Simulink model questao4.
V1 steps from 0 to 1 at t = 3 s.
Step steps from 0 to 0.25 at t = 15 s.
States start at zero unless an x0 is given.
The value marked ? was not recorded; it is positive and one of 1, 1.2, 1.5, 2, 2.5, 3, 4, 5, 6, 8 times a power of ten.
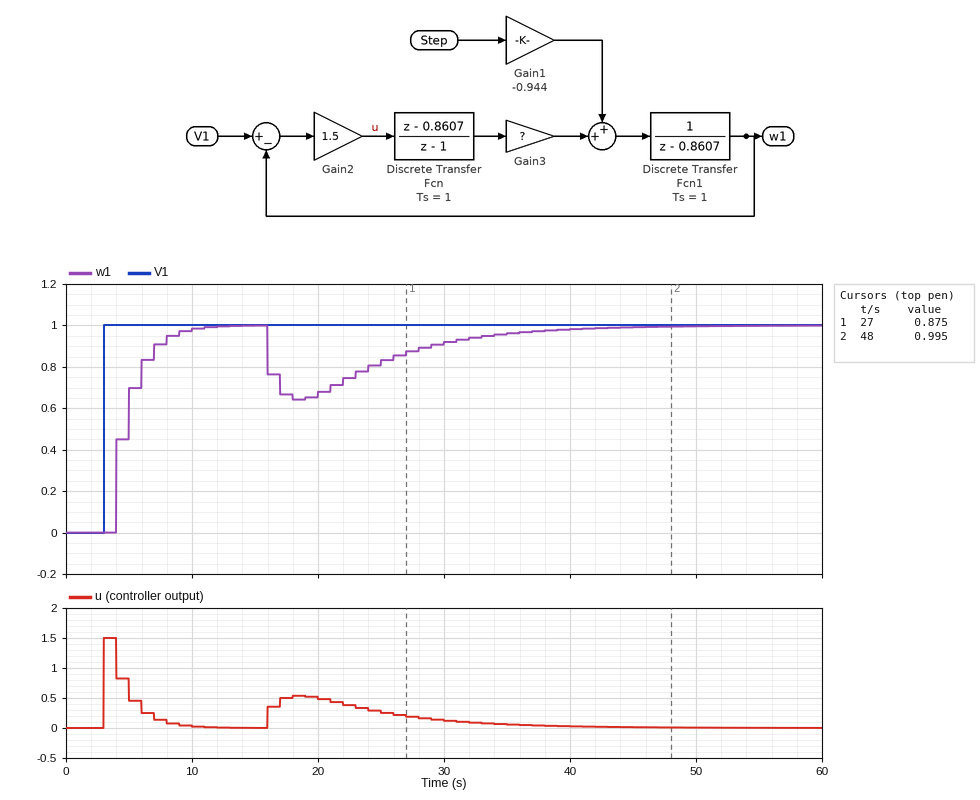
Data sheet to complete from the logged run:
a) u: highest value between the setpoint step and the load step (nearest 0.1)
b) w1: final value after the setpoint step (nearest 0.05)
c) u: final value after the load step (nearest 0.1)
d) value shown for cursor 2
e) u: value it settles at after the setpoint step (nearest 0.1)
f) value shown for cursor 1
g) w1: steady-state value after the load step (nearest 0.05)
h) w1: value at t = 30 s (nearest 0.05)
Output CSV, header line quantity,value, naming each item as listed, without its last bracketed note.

quantity,value
u: highest value between the setpoint step and the load step,1.5
w1: final value after the setpoint step,1.00
u: final value after the load step,0.0
value shown for cursor 2,0.995
u: value it settles at after the setpoint step,0.0
value shown for cursor 1,0.875
w1: steady-state value after the load step,1.00
w1: value at t = 30 s,0.90
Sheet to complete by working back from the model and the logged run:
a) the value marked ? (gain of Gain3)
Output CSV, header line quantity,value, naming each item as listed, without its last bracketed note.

quantity,value
the value marked ?,0.3
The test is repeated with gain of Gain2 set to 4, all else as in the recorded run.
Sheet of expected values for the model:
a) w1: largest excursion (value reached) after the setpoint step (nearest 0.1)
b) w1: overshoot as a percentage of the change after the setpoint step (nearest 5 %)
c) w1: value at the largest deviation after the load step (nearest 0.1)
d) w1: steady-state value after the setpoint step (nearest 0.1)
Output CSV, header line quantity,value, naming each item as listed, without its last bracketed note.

quantity,value
w1: largest excursion (value reached) after the setpoint step,1.2
w1: overshoot as a percentage of the change after the setpoint step,20 %
w1: value at the largest deviation after the load step,0.8
w1: steady-state value after the setpoint step,1.0
